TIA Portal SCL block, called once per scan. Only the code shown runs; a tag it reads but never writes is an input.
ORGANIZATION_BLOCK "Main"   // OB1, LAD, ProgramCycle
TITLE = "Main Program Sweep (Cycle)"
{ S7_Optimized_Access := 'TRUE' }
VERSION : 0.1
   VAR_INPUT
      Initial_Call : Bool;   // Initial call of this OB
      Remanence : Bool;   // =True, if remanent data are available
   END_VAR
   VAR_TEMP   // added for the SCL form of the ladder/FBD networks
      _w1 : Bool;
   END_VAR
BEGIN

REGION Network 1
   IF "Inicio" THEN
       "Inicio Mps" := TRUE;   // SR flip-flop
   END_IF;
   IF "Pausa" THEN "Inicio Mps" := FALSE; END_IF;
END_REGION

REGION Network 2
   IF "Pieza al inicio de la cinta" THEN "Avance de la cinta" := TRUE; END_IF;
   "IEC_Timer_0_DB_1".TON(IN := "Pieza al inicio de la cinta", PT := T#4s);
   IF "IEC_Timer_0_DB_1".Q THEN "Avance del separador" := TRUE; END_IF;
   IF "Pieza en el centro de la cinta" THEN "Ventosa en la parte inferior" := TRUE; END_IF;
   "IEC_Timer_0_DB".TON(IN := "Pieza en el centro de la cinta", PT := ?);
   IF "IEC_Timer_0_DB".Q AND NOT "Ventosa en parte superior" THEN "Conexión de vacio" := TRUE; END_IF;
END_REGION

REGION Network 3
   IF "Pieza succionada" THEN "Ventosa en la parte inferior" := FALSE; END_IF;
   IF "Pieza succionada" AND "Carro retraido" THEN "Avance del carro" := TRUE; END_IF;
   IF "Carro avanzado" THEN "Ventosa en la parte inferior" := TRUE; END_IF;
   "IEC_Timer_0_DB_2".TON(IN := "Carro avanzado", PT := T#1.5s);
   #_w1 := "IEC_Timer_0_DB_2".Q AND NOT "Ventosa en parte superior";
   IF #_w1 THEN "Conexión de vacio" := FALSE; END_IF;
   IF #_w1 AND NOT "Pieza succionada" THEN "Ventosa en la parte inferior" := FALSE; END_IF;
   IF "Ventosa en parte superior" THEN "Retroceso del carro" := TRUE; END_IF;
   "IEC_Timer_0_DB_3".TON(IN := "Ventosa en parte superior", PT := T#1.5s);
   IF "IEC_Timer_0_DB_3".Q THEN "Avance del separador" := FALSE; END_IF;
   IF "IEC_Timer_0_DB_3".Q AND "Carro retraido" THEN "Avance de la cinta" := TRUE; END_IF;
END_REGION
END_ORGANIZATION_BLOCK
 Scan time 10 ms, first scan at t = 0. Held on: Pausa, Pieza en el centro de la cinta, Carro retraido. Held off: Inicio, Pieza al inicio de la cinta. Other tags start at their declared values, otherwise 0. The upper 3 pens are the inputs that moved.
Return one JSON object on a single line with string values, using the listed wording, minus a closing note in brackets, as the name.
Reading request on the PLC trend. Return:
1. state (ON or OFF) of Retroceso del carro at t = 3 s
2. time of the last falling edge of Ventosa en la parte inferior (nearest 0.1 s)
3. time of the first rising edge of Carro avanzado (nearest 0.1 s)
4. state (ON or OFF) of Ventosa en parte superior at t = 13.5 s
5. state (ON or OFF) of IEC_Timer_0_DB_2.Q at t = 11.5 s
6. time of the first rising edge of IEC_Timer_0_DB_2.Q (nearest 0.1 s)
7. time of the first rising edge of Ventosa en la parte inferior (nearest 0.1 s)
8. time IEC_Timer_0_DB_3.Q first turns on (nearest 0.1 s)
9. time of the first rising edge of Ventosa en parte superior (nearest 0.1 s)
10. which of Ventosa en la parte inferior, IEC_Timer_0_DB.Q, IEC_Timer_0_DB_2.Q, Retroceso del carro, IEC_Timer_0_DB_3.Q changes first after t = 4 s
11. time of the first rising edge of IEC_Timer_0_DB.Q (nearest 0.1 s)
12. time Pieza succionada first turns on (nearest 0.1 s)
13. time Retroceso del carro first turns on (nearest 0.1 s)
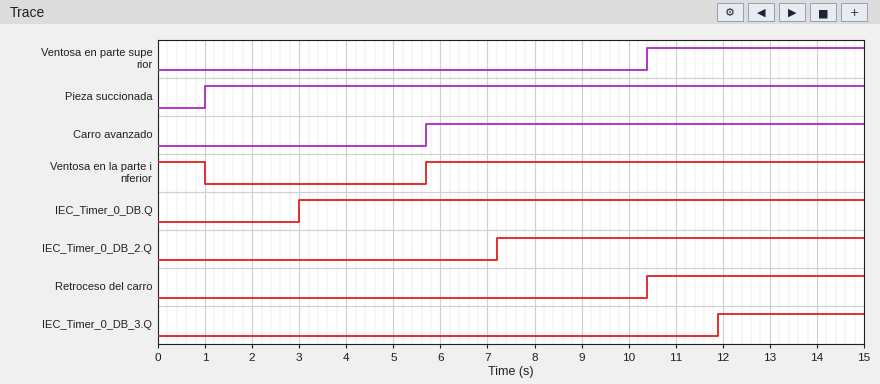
{"state (ON or OFF) of Retroceso del carro at t = 3 s": "OFF", "time of the last falling edge of Ventosa en la parte inferior": "1.0 s", "time of the first rising edge of Carro avanzado": "5.7 s", "state (ON or OFF) of Ventosa en parte superior at t = 13.5 s": "ON", "state (ON or OFF) of IEC_Timer_0_DB_2.Q at t = 11.5 s": "ON", "time of the first rising edge of IEC_Timer_0_DB_2.Q": "7.2 s", "time of the first rising edge of Ventosa en la parte inferior": "5.7 s", "time IEC_Timer_0_DB_3.Q first turns on": "11.9 s", "time of the first rising edge of Ventosa en parte superior": "10.4 s", "which of Ventosa en la parte inferior, IEC_Timer_0_DB.Q, IEC_Timer_0_DB_2.Q, Retroceso del carro, IEC_Timer_0_DB_3.Q changes first after t = 4 s": "Ventosa en la parte inferior", "time of the first rising edge of IEC_Timer_0_DB.Q": "3.0 s", "time Pieza succionada first turns on": "1.0 s", "time Retroceso del carro first turns on": "10.4 s"}
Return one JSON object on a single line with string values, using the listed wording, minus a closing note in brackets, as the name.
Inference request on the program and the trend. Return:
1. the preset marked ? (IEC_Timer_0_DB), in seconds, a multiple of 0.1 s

{"the preset marked ? (IEC_Timer_0_DB), in seconds, a multiple of 0.1 s": "3.0 s"}
